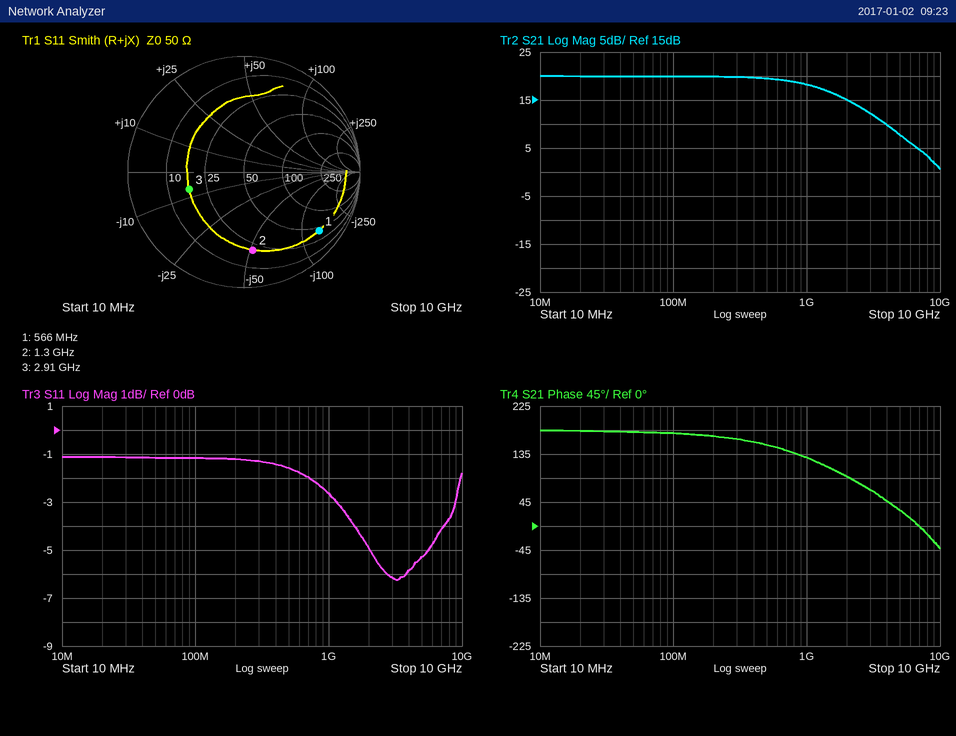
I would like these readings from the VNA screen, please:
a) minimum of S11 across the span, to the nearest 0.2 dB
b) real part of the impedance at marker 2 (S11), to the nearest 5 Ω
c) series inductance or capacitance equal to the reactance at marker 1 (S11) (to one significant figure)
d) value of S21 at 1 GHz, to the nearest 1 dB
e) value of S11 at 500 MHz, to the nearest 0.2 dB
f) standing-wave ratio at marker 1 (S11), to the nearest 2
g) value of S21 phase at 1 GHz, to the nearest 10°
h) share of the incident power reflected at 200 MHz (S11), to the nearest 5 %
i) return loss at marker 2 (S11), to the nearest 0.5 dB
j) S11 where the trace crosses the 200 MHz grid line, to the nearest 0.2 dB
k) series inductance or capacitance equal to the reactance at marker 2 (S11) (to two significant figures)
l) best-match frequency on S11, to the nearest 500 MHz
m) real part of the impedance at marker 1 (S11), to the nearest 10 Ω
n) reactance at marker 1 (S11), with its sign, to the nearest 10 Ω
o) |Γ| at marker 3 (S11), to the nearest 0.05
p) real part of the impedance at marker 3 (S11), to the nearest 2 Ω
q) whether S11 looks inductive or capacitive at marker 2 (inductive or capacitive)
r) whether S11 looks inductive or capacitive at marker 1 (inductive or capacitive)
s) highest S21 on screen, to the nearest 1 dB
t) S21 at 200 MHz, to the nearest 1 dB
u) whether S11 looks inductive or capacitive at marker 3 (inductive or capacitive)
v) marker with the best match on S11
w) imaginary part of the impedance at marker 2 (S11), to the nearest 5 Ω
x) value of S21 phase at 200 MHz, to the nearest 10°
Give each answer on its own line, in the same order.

-6.2 dB
20 Ω
2 pF
18 dB
-1.6 dB
10
130°
75 %
3.5 dB
-1.2 dB
2.4 pF
3.0 GHz
40 Ω
-130 Ω
0.50
18 Ω
capacitive
capacitive
20 dB
20 dB
capacitive
marker 3
-50 Ω
170°
